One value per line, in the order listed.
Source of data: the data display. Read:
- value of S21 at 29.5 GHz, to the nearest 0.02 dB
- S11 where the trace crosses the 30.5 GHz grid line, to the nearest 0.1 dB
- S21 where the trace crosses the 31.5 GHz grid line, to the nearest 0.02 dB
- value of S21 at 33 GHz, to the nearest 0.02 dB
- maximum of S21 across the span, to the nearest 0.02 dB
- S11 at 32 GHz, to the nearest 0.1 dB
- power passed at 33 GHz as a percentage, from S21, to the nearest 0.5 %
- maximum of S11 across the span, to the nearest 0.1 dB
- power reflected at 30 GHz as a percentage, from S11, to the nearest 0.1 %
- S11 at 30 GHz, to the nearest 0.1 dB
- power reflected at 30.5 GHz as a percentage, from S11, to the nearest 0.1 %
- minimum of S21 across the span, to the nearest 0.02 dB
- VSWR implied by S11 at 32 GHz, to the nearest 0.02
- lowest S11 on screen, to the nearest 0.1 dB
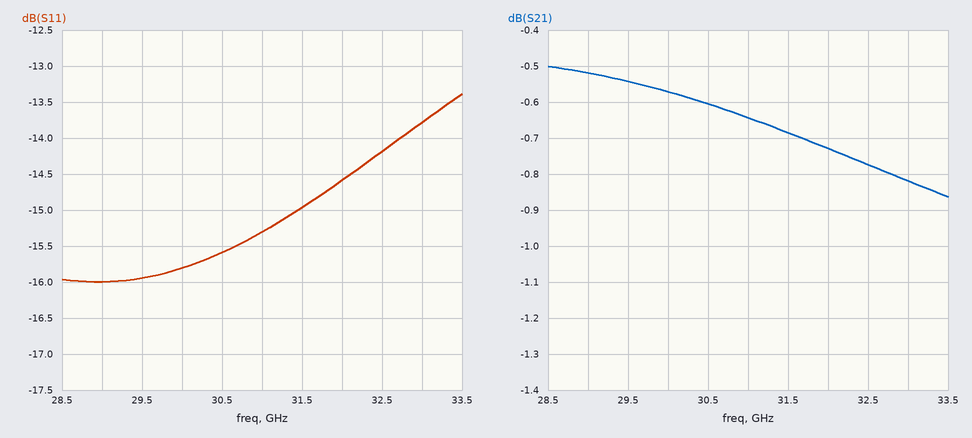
-0.54 dB
-15.6 dB
-0.68 dB
-0.82 dB
-0.50 dB
-14.6 dB
83.0 %
-13.4 dB
2.6 %
-15.8 dB
2.8 %
-0.86 dB
1.46
-16.0 dB
